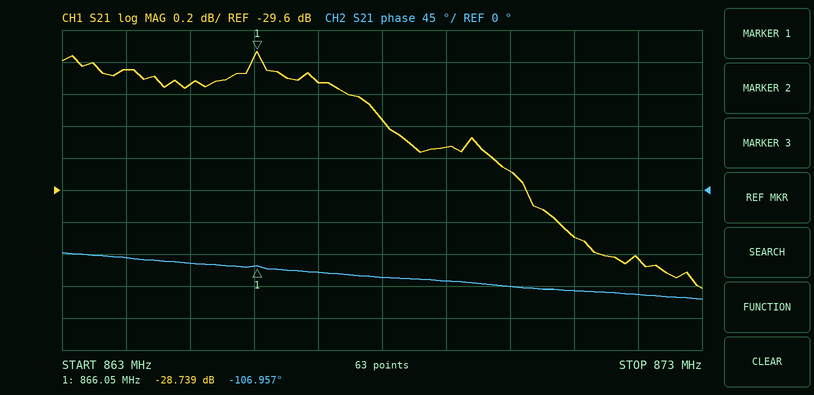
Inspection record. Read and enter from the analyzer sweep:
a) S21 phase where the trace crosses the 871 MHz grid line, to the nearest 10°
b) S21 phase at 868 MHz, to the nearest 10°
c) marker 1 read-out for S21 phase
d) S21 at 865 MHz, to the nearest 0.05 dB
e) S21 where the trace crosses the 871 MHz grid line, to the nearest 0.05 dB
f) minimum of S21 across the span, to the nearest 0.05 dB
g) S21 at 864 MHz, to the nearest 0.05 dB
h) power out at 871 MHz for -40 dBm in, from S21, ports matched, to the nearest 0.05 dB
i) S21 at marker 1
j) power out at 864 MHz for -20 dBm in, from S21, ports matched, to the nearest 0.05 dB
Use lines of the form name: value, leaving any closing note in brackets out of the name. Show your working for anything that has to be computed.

S21 phase where the trace crosses the 871 MHz grid line, to the nearest 10°: -140°
S21 phase at 868 MHz, to the nearest 10°: -120°
marker 1 read-out for S21 phase: -106.957°
S21 at 865 MHz, to the nearest 0.05 dB: -28.95 dB
S21 where the trace crosses the 871 MHz grid line, to the nearest 0.05 dB: -29.90 dB
minimum of S21 across the span, to the nearest 0.05 dB: -30.20 dB
S21 at 864 MHz, to the nearest 0.05 dB: -28.85 dB
power out at 871 MHz for -40 dBm in, from S21, ports matched, to the nearest 0.05 dB: -40 dBm + (-29.90 dB) = -69.90 dBm
S21 at marker 1: -28.739 dB
power out at 864 MHz for -20 dBm in, from S21, ports matched, to the nearest 0.05 dB: -20 dBm + (-28.85 dB) = -48.85 dBm
